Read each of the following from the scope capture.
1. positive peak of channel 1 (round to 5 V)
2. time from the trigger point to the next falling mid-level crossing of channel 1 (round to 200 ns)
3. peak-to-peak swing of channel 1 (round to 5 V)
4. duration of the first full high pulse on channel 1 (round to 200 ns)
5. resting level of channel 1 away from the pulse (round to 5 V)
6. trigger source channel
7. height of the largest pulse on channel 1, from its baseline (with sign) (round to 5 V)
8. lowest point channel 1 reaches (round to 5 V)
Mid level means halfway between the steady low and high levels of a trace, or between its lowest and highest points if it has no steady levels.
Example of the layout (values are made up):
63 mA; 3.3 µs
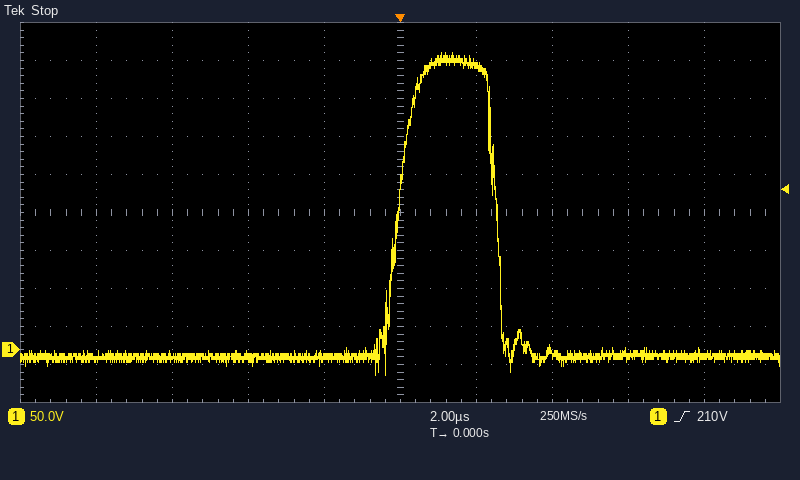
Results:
390 V; 2.6 µs; 425 V; 2.6 µs; -10 V; channel 1; +400 V; -35 V
